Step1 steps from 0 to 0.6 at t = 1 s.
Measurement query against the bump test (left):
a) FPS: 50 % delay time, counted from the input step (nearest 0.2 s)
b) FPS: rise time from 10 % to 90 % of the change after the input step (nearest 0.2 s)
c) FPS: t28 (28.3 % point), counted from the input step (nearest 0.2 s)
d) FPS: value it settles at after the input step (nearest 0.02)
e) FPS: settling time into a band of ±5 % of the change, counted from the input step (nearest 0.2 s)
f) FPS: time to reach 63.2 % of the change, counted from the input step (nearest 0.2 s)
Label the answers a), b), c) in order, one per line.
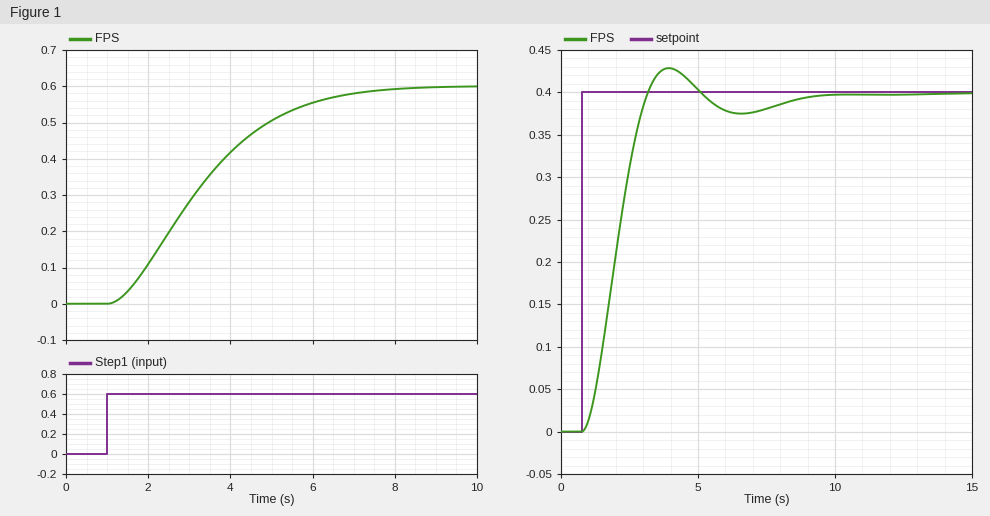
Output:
a) 2.2 s
b) 4.0 s
c) 1.4 s
d) 0.60
e) 5.6 s
f) 2.6 s
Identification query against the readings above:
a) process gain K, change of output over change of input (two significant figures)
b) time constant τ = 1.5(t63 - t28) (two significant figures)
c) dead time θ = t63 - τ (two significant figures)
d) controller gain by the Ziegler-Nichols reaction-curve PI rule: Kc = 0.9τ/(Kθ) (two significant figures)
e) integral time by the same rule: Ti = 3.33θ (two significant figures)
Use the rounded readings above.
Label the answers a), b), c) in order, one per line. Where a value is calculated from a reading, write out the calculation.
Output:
a) (0.6 - 0) / 0.6 = 1.0
b) 1.5 × (2.6 - 1.4) = 1.8 s
c) 2.6 - 1.8 = 0.80 s
d) 0.9 × 1.8 / (1 × 0.8) = 2.0
e) 3.33 × 0.8 = 2.7 s
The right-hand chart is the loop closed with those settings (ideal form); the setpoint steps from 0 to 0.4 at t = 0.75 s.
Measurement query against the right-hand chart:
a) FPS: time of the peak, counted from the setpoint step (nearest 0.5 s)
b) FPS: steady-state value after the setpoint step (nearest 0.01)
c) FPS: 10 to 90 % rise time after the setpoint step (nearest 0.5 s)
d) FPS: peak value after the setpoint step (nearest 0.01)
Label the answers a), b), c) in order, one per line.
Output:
a) 3.0 s
b) 0.40
c) 1.5 s
d) 0.43
